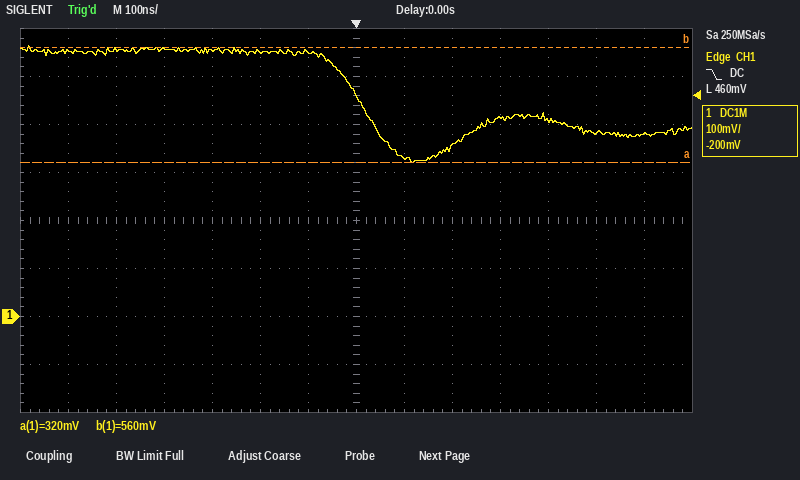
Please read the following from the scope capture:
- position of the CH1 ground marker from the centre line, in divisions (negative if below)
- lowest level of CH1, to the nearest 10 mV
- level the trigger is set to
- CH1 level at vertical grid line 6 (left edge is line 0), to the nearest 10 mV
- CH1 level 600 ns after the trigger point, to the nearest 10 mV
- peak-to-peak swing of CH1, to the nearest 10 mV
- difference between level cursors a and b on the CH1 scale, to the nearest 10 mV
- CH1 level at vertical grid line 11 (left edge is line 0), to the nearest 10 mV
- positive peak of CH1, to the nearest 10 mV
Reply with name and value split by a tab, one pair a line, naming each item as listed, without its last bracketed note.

position of the CH1 ground marker from the centre line, in divisions	-2.0 div
lowest level of CH1, to the nearest 10 mV	320 mV
level the trigger is set to	460 mV
CH1 level at vertical grid line 6 (left edge is line 0), to the nearest 10 mV	550 mV
CH1 level 600 ns after the trigger point, to the nearest 10 mV	380 mV
peak-to-peak swing of CH1, to the nearest 10 mV	240 mV
difference between level cursors a and b on the CH1 scale, to the nearest 10 mV	240 mV
CH1 level at vertical grid line 11 (left edge is line 0), to the nearest 10 mV	410 mV
positive peak of CH1, to the nearest 10 mV	560 mV
